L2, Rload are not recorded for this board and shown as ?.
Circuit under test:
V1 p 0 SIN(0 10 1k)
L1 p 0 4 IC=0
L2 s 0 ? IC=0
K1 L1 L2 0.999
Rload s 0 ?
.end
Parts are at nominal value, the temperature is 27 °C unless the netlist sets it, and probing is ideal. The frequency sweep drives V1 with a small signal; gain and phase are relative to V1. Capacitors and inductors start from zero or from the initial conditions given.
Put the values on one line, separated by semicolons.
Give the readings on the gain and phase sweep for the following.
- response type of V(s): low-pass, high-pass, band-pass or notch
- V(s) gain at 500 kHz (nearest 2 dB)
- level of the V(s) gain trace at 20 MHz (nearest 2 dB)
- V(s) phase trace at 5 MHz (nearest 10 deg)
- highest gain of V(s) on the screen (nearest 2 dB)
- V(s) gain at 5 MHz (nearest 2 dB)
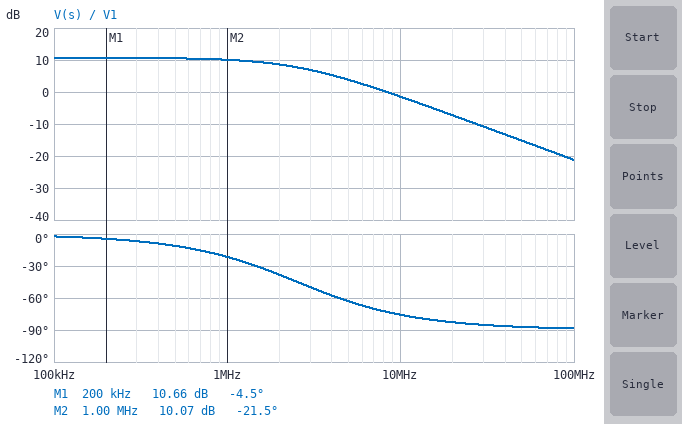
low-pass; 10 dB; -8 dB; -60 deg; 10 dB; 4 dB
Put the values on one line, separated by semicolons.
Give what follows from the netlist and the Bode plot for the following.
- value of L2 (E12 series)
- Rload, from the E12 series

47 H; 1.5 MΩ
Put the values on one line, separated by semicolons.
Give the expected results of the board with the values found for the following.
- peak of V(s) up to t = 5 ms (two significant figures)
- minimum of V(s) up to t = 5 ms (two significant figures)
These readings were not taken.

34 V; -34 V
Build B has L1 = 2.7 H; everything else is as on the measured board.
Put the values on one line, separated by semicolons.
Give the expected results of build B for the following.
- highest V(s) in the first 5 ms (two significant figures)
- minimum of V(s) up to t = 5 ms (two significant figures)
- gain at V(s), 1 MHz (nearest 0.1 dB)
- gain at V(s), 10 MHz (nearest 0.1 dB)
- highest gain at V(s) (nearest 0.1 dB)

42 V; -42 V; 11.8 dB; 0.2 dB; 12.4 dB
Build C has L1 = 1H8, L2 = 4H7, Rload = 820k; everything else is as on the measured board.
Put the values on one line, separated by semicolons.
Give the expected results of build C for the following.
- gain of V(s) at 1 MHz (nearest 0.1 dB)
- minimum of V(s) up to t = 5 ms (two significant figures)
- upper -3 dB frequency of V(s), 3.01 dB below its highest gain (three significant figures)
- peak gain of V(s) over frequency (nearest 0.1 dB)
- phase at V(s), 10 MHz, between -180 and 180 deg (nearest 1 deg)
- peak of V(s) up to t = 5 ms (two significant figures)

4.1 dB; -16 V; 13.9 MHz; 4.2 dB; -36 deg; 16 V
